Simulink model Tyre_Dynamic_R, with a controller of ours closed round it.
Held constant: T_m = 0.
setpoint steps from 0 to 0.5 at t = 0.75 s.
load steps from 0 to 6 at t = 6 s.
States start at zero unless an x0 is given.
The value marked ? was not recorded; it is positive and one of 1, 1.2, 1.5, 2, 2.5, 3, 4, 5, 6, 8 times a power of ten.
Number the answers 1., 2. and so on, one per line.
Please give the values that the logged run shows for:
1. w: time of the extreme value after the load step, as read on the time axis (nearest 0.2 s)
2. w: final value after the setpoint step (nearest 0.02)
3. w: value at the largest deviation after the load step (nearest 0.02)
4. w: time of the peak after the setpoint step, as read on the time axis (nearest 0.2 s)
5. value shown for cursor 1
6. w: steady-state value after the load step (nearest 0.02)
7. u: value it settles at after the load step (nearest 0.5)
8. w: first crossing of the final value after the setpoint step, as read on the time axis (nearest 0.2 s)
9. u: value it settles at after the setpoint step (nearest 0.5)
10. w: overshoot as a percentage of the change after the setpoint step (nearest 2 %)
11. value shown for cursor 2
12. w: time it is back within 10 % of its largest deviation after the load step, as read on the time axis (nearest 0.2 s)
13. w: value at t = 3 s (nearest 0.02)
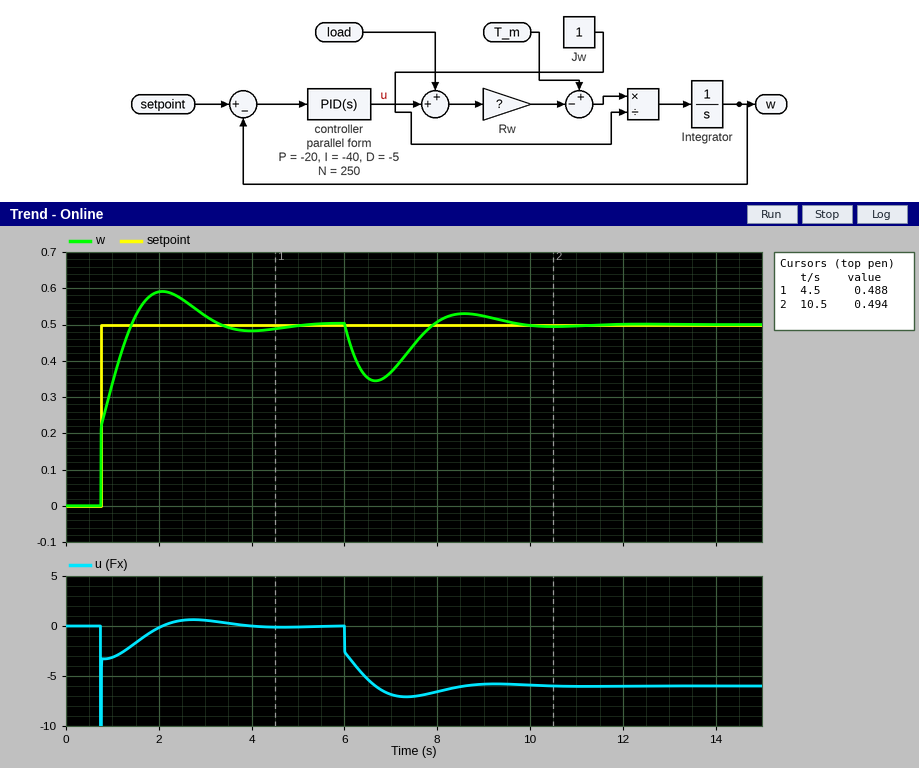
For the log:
1. 6.6 s
2. 0.50
3. 0.34
4. 2.0 s
5. 0.488
6. 0.50
7. -6.0
8. 1.4 s
9. 0.0
10. 18 %
11. 0.494
12. 9.2 s
13. 0.52
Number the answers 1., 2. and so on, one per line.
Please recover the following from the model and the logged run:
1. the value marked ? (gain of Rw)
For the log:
1. 0.15
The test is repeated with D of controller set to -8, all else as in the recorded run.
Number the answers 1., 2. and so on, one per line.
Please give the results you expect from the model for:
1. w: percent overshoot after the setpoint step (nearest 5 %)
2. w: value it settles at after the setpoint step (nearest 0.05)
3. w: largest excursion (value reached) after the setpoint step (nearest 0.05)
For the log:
1. 15 %
2. 0.50
3. 0.60
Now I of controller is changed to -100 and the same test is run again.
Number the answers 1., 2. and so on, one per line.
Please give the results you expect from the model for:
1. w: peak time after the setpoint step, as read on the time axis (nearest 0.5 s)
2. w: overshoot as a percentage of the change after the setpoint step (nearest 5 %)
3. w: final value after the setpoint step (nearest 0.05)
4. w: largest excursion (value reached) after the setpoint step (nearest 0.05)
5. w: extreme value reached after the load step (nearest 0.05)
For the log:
1. 1.5 s
2. 25 %
3. 0.50
4. 0.65
5. 0.40
